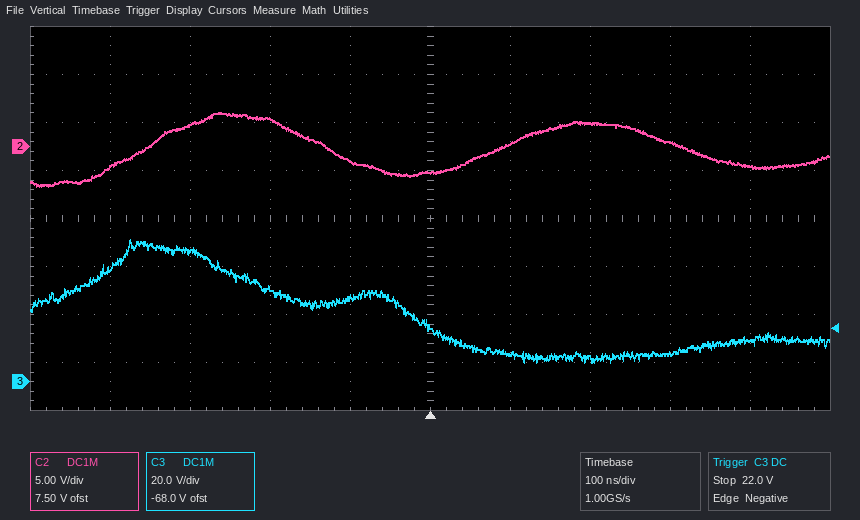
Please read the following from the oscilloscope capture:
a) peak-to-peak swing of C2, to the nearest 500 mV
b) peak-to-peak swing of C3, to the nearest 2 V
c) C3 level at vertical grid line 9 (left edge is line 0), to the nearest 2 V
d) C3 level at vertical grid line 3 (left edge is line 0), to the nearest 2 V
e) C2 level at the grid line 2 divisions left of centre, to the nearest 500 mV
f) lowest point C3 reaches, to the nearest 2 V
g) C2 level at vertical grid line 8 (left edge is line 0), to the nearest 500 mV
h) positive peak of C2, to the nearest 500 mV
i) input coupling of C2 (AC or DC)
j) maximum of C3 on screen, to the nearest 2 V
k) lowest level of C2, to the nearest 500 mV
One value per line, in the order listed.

7.5 V
52 V
18 V
38 V
3.0 V
8 V
500 mV
3.5 V
DC
60 V
-4.0 V
